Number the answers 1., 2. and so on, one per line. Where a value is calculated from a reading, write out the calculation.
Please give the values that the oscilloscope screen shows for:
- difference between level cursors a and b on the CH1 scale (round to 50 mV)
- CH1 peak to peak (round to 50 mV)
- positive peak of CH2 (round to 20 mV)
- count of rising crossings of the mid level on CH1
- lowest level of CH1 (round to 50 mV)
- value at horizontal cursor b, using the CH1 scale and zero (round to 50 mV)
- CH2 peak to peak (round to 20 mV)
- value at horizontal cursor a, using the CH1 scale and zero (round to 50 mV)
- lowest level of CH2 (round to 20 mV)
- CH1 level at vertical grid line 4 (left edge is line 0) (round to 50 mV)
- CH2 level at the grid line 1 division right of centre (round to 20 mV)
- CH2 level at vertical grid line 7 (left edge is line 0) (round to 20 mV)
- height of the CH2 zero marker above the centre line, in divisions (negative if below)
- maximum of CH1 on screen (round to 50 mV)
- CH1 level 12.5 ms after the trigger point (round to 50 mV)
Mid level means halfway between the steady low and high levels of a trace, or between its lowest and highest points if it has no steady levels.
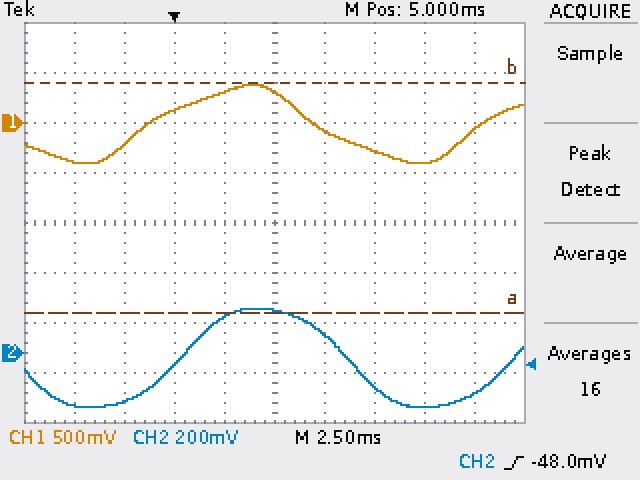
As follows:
1. 2.30 V
2. 400 mV − (-400 mV) = 800 mV
3. 180 mV
4. 2
5. -400 mV
6. 400 mV
7. 180 mV − (-220 mV) = 400 mV
8. -1.90 V
9. -220 mV
10. 300 mV
11. 80 mV
12. -140 mV
13. -2.6 div
14. 400 mV
15. -400 mV
